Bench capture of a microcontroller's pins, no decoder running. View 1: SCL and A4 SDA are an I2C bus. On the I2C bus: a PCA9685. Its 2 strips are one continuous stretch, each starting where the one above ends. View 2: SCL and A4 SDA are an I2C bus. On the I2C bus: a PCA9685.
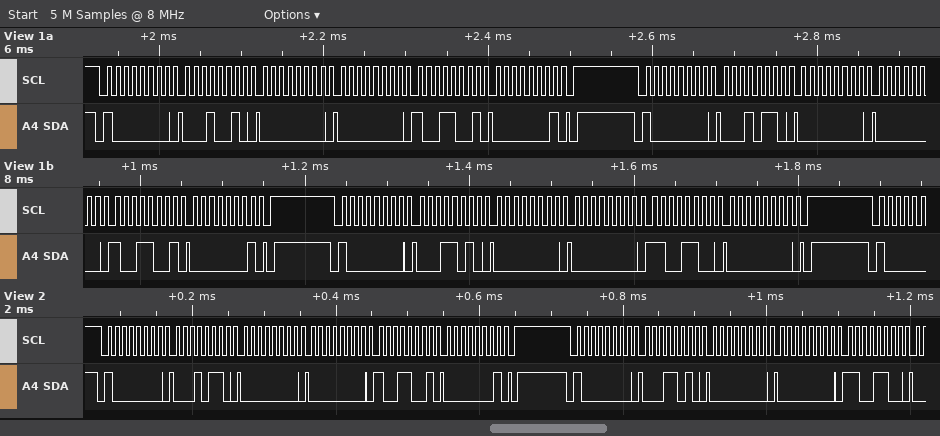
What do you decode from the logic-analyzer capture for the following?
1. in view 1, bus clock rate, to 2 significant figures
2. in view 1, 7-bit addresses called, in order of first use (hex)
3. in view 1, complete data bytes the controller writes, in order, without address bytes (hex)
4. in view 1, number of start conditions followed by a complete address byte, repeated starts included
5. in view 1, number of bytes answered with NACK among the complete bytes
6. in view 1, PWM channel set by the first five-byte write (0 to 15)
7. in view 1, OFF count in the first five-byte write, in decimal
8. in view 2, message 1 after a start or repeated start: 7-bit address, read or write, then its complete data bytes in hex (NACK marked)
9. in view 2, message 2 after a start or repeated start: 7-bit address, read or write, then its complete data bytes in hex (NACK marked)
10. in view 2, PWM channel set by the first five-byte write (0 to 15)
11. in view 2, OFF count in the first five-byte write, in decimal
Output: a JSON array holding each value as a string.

["100 kHz", "0x40", "12 00 00 99 01 16 00 00 99 01 1A 00 00 CC 00", "3", "0", "3", "409", "0x40 write: 16 00 00 99 01", "0x40 write: 1A 00 00 CC", "4", "409"]
